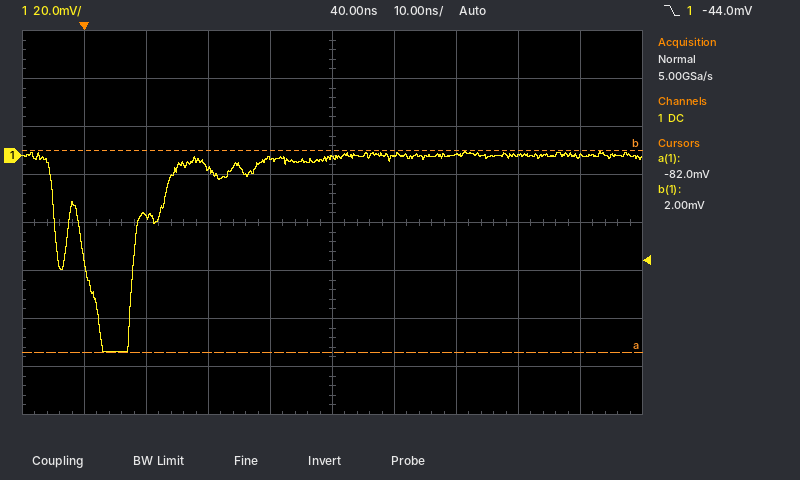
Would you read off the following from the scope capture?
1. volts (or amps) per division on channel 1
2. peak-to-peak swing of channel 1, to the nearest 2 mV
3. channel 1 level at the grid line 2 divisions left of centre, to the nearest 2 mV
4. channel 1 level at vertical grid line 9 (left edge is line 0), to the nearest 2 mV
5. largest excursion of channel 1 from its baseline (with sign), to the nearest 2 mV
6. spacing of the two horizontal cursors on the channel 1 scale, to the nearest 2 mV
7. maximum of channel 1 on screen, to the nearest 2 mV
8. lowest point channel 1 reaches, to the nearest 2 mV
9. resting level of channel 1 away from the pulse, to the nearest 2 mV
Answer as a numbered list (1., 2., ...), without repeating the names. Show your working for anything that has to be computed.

1. 20 mV
2. 2 mV − (-82 mV) = 84 mV
3. -6 mV
4. 0 mV
5. -82 mV − (0 mV) = -82 mV
6. 84 mV
7. 2 mV
8. -82 mV
9. 0 mV
